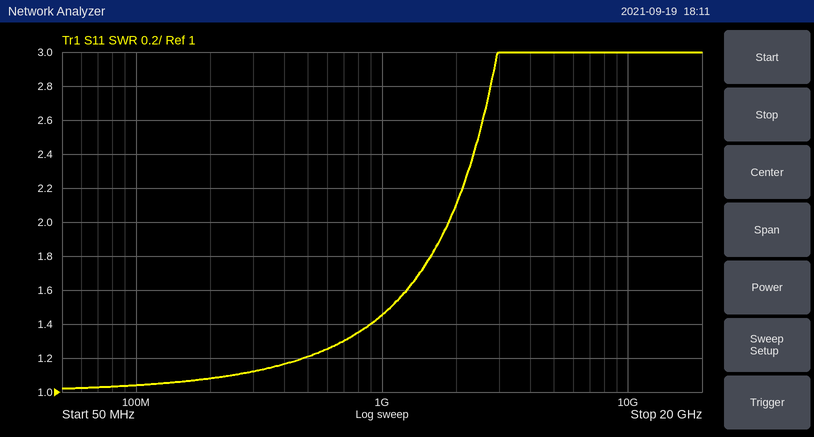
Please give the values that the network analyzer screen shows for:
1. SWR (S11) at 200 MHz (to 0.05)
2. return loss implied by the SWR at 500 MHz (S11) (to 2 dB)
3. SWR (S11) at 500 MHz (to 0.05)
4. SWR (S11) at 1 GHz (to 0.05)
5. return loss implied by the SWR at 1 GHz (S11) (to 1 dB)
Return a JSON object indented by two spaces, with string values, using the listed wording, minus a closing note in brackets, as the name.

{
  "SWR (S11) at 200 MHz": "1.10",
  "return loss implied by the SWR at 500 MHz (S11)": "20 dB",
  "SWR (S11) at 500 MHz": "1.20",
  "SWR (S11) at 1 GHz": "1.45",
  "return loss implied by the SWR at 1 GHz (S11)": "15 dB"
}
